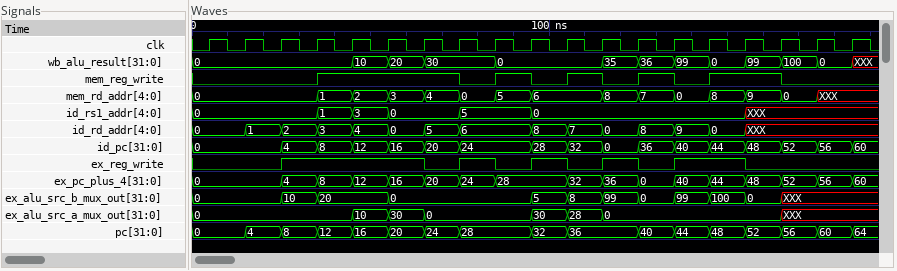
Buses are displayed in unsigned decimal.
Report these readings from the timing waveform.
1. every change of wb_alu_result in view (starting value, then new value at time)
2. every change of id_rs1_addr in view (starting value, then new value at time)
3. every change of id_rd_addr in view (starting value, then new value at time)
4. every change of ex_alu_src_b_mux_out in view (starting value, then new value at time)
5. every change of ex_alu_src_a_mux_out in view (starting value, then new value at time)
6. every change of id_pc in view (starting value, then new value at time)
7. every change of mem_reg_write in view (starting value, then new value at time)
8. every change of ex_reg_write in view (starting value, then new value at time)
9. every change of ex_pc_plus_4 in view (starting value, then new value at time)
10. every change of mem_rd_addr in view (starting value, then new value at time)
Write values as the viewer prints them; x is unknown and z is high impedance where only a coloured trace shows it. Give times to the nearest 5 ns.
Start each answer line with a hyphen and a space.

- 0, 10 at 45 ns, 20 at 55 ns, 30 at 65 ns, 0 at 85 ns, 35 at 115 ns, 36 at 125 ns, 99 at 135 ns, 0 at 145 ns, 99 at 155 ns, 100 at 165 ns, 0 at 175 ns, XXX at 185 ns
- 0, 1 at 35 ns, 3 at 45 ns, 0 at 55 ns, 5 at 75 ns, 0 at 95 ns, XXX at 155 ns
- 0, 1 at 15 ns, 2 at 25 ns, 3 at 35 ns, 4 at 45 ns, 0 at 55 ns, 5 at 65 ns, 6 at 75 ns, 8 at 95 ns, 7 at 105 ns, 0 at 115 ns, 8 at 125 ns, 9 at 135 ns, 0 at 145 ns, XXX at 155 ns
- 0, 10 at 25 ns, 20 at 35 ns, 0 at 55 ns, 5 at 95 ns, 8 at 105 ns, 99 at 115 ns, 0 at 125 ns, 99 at 135 ns, 100 at 145 ns, 0 at 155 ns, XXX at 165 ns
- 0, 10 at 45 ns, 30 at 55 ns, 0 at 65 ns, 30 at 95 ns, 28 at 105 ns, 0 at 115 ns, XXX at 165 ns
- 0, 4 at 25 ns, 8 at 35 ns, 12 at 45 ns, 16 at 55 ns, 20 at 65 ns, 24 at 75 ns, 28 at 95 ns, 32 at 105 ns, 0 at 115 ns, 36 at 125 ns, 40 at 135 ns, 44 at 145 ns, 48 at 155 ns, 52 at 165 ns, 56 at 175 ns, 60 at 185 ns
- 0, 1 at 35 ns, 0 at 75 ns, 1 at 85 ns, 0 at 95 ns, 1 at 105 ns, 0 at 115 ns, 1 at 125 ns, 0 at 135 ns, 1 at 145 ns, 0 at 165 ns
- 0, 1 at 25 ns, 0 at 65 ns, 1 at 75 ns, 0 at 85 ns, 1 at 95 ns, 0 at 105 ns, 1 at 115 ns, 0 at 125 ns, 1 at 135 ns, 0 at 155 ns
- 0, 4 at 25 ns, 8 at 35 ns, 12 at 45 ns, 16 at 55 ns, 20 at 65 ns, 24 at 75 ns, 28 at 85 ns, 32 at 105 ns, 36 at 115 ns, 0 at 125 ns, 40 at 135 ns, 44 at 145 ns, 48 at 155 ns, 52 at 165 ns, 56 at 175 ns, 60 at 185 ns
- 0, 1 at 35 ns, 2 at 45 ns, 3 at 55 ns, 4 at 65 ns, 0 at 75 ns, 5 at 85 ns, 6 at 95 ns, 8 at 115 ns, 7 at 125 ns, 0 at 135 ns, 8 at 145 ns, 9 at 155 ns, 0 at 165 ns, XXX at 175 ns
